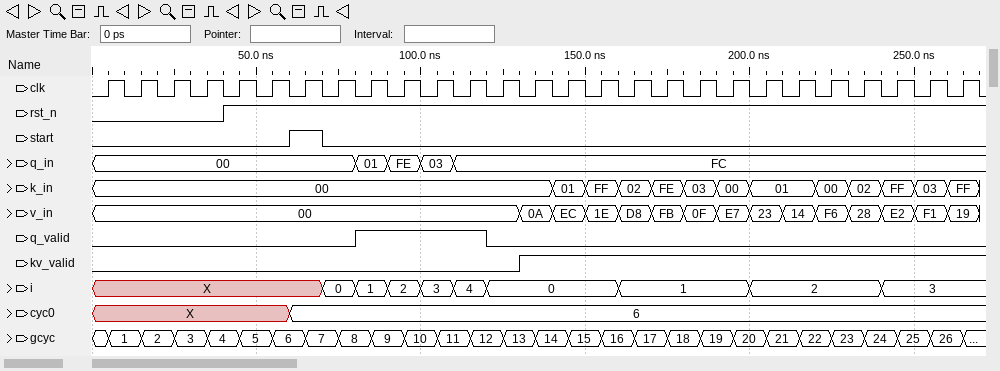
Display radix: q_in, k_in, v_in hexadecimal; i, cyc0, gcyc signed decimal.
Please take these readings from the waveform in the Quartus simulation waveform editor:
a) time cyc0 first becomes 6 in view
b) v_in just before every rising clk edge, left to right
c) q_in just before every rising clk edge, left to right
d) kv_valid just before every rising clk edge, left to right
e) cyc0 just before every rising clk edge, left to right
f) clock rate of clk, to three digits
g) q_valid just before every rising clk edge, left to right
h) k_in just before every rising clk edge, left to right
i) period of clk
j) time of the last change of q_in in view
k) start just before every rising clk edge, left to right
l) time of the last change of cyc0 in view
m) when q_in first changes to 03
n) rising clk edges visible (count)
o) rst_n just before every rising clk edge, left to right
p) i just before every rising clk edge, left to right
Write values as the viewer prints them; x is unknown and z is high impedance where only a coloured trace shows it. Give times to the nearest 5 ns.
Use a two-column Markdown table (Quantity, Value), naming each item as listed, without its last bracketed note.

| Quantity | Value |
|---|---|
| time cyc0 first becomes 6 in view | 60 ns |
| v_in just before every rising clk edge, left to right | 00, 00, 00, 00, 00, 00, 00, 00, 00, 00, 00, 00, 00, 0A, EC, 1E, D8, FB, 0F, E7, 23, 14, F6, 28, E2, F1, 19 |
| q_in just before every rising clk edge, left to right | 00, 00, 00, 00, 00, 00, 00, 00, 01, FE, 03, FC, FC, FC, FC, FC, FC, FC, FC, FC, FC, FC, FC, FC, FC, FC, FC |
| kv_valid just before every rising clk edge, left to right | 0 0 0 0 0 0 0 0 0 0 0 0 0 1 1 1 1 1 1 1 1 1 1 1 1 1 1 |
| cyc0 just before every rising clk edge, left to right | X, X, X, X, X, X, 6, 6, 6, 6, 6, 6, 6, 6, 6, 6, 6, 6, 6, 6, 6, 6, 6, 6, 6, 6, 6 |
| clock rate of clk, to three digits | 100 MHz |
| q_valid just before every rising clk edge, left to right | 0 0 0 0 0 0 0 0 1 1 1 1 0 0 0 0 0 0 0 0 0 0 0 0 0 0 0 |
| k_in just before every rising clk edge, left to right | 00, 00, 00, 00, 00, 00, 00, 00, 00, 00, 00, 00, 00, 00, 01, FF, 02, FE, 03, 00, 01, 01, 00, 02, FF, 03, FF |
| period of clk | 10 ns |
| time of the last change of q_in in view | 110 ns |
| start just before every rising clk edge, left to right | 0 0 0 0 0 0 1 0 0 0 0 0 0 0 0 0 0 0 0 0 0 0 0 0 0 0 0 |
| time of the last change of cyc0 in view | 60 ns |
| when q_in first changes to 03 | 100 ns |
| rising clk edges visible | 27 |
| rst_n just before every rising clk edge, left to right | 0 0 0 0 1 1 1 1 1 1 1 1 1 1 1 1 1 1 1 1 1 1 1 1 1 1 1 |
| i just before every rising clk edge, left to right | X, X, X, X, X, X, X, 0, 1, 2, 3, 4, 0, 0, 0, 0, 1, 1, 1, 1, 2, 2, 2, 2, 3, 3, 3 |
